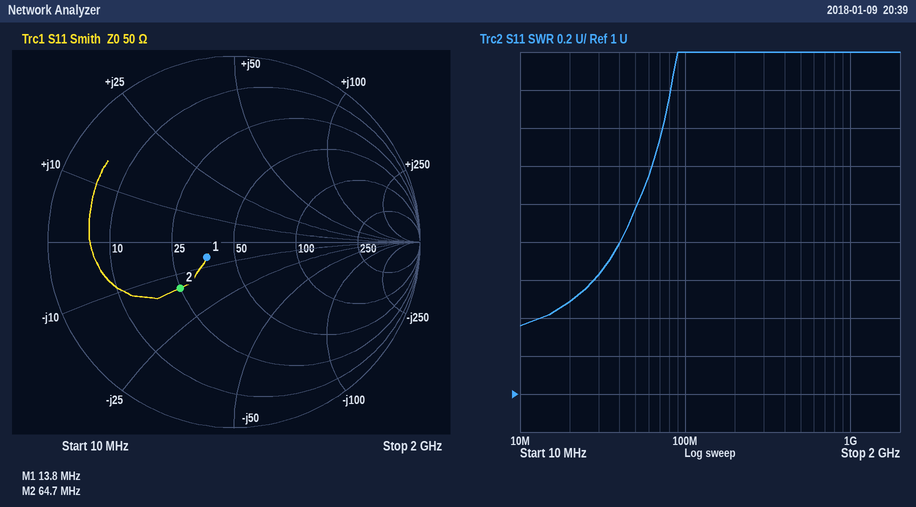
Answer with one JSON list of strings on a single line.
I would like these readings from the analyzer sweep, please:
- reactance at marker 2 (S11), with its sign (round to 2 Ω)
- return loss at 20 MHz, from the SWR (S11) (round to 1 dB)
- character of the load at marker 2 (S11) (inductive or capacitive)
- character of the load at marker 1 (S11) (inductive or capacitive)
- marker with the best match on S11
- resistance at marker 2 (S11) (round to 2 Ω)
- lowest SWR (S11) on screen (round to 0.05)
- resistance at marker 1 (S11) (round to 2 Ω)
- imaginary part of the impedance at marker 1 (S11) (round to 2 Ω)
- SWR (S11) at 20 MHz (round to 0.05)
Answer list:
["-14 Ω", "14 dB", "capacitive", "capacitive", "marker 1", "24 Ω", "1.35", "36 Ω", "-6 Ω", "1.50"]
